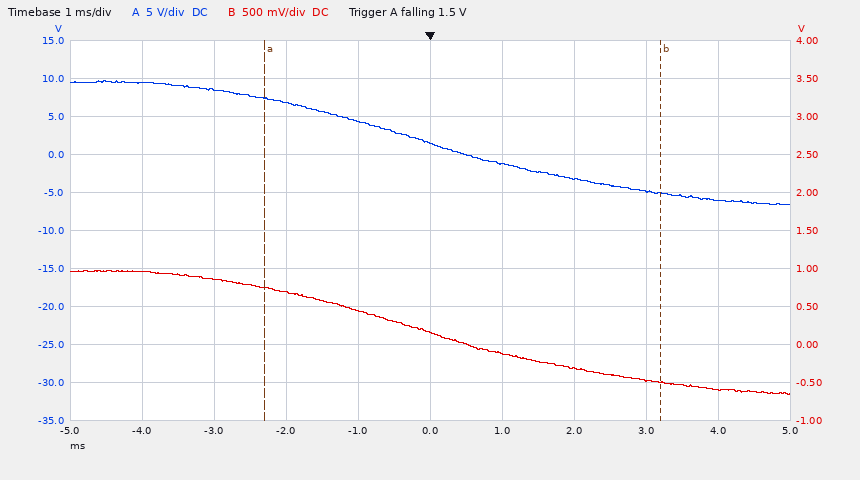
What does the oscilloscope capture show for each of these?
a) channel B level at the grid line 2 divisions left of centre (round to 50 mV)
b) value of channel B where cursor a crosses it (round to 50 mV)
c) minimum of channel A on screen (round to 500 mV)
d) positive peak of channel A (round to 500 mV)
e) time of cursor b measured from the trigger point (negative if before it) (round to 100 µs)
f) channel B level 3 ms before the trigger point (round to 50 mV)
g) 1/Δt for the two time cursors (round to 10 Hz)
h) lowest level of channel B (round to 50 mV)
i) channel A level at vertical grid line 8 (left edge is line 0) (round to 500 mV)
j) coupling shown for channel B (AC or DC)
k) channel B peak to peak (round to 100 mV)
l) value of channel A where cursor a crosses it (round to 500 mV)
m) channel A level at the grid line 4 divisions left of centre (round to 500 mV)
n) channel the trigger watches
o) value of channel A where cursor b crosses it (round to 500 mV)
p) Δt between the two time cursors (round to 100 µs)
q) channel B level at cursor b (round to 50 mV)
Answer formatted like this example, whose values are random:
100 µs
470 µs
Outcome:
700 mV
750 mV
-6.5 V
9.5 V
+3.2 ms
850 mV
180 Hz
-650 mV
-5.0 V
DC
1.60 V
7.5 V
9.5 V
channel A
-5.0 V
5.5 ms
-500 mV
